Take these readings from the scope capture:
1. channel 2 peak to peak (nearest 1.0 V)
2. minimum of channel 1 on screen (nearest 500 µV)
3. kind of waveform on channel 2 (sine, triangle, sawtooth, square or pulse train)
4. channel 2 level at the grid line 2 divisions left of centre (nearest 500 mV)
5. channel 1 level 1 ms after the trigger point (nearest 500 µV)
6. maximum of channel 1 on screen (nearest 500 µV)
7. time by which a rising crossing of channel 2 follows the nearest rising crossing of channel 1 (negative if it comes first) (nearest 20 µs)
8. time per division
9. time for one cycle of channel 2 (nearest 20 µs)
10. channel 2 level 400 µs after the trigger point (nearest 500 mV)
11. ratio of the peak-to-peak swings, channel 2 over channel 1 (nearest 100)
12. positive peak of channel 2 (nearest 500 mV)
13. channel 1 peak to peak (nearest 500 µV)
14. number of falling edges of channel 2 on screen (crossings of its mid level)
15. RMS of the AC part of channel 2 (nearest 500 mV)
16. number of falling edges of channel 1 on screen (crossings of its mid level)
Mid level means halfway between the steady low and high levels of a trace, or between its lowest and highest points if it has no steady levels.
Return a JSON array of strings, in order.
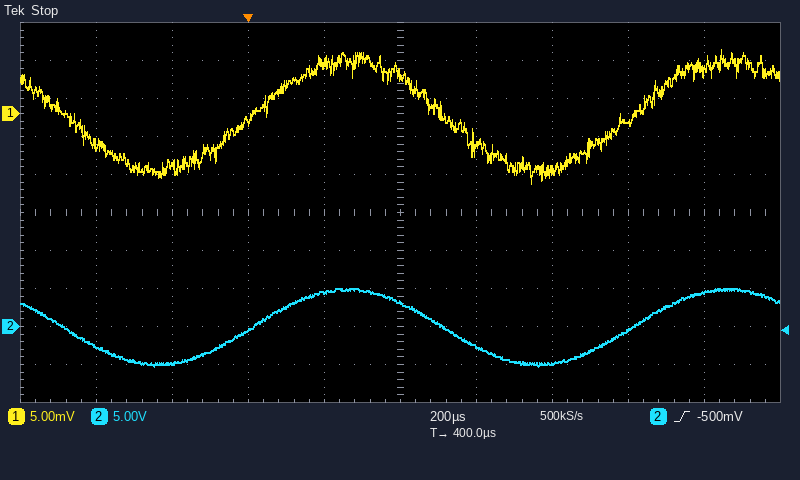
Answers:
["10.0 V", "-9.0 mV", "sine", "-500 mV", "-1.0 mV", "8.5 mV", "0 µs", "200 µs", "1.00 ms", "3.0 V", "600", "5.0 V", "17.5 mV", "2", "3.5 V", "2"]
